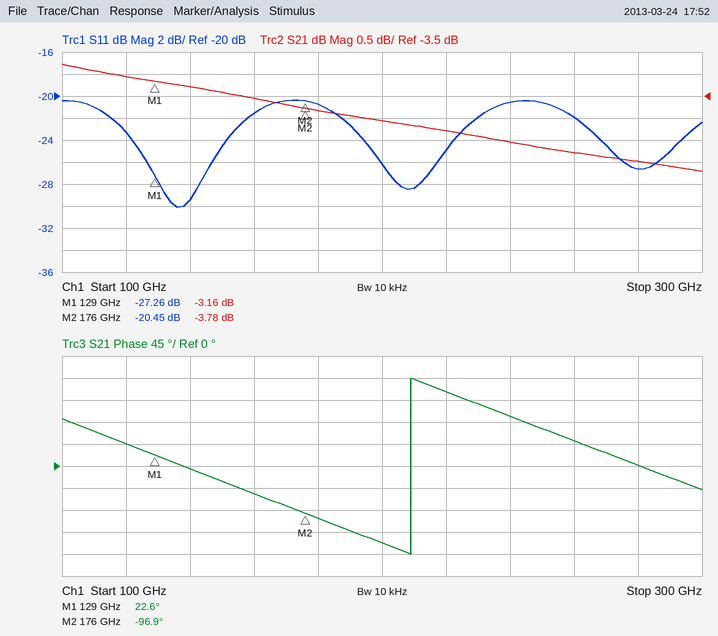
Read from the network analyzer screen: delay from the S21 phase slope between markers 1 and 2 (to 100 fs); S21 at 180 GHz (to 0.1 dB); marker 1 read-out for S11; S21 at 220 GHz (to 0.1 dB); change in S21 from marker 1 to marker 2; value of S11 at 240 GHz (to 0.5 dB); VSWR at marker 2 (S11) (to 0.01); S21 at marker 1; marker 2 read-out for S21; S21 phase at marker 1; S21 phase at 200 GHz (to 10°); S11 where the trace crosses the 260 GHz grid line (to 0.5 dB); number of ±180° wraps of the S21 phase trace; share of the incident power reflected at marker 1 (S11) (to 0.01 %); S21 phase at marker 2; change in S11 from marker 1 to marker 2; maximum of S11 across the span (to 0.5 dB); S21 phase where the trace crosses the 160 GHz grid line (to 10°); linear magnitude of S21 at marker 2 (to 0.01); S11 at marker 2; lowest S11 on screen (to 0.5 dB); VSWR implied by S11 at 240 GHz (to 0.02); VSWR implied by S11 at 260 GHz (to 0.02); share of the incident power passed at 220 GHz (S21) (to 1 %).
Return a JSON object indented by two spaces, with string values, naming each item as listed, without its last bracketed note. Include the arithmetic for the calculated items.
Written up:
{
  "delay from the S21 phase slope between markers 1 and 2": "−(-96.9° − (22.6°))/(360° × 47 GHz) ≈ 7.1 ps",
  "S21 at 180 GHz": "-3.8 dB",
  "marker 1 read-out for S11": "-27.26 dB",
  "S21 at 220 GHz": "-4.3 dB",
  "change in S21 from marker 1 to marker 2": "-3.78 − (-3.16) = -0.62 dB",
  "value of S11 at 240 GHz": "-20.5 dB",
  "VSWR at marker 2 (S11)": "(1 + 0.0950)/(1 − 0.0950) ≈ 1.21",
  "S21 at marker 1": "-3.16 dB",
  "marker 2 read-out for S21": "-3.78 dB",
  "S21 phase at marker 1": "22.6°",
  "S21 phase at 200 GHz": "-160°",
  "S11 where the trace crosses the 260 GHz grid line": "-22.0 dB",
  "number of ±180° wraps of the S21 phase trace": "1",
  "share of the incident power reflected at marker 1 (S11)": "10^(-27.26/10) ≈ 0.19 %",
  "S21 phase at marker 2": "-96.9°",
  "change in S11 from marker 1 to marker 2": "-20.45 − (-27.26) = 6.81 dB",
  "maximum of S11 across the span": "-20.5 dB",
  "S21 phase where the trace crosses the 160 GHz grid line": "-60°",
  "linear magnitude of S21 at marker 2": "10^(-3.78/20) ≈ 0.65",
  "S11 at marker 2": "-20.45 dB",
  "lowest S11 on screen": "-30.0 dB",
  "VSWR implied by S11 at 240 GHz": "|Γ| = 10^(-20.5/20) = 0.0944; VSWR = (1 + 0.0944)/(1 − 0.0944) ≈ 1.21, so 1.20 to the nearest 0.02",
  "VSWR implied by S11 at 260 GHz": "|Γ| = 10^(-22/20) = 0.0794; VSWR = (1 + 0.0794)/(1 − 0.0794) ≈ 1.17, so 1.18 to the nearest 0.02",
  "share of the incident power passed at 220 GHz (S21)": "10^(-4.3/10) ≈ 37 %"
}
